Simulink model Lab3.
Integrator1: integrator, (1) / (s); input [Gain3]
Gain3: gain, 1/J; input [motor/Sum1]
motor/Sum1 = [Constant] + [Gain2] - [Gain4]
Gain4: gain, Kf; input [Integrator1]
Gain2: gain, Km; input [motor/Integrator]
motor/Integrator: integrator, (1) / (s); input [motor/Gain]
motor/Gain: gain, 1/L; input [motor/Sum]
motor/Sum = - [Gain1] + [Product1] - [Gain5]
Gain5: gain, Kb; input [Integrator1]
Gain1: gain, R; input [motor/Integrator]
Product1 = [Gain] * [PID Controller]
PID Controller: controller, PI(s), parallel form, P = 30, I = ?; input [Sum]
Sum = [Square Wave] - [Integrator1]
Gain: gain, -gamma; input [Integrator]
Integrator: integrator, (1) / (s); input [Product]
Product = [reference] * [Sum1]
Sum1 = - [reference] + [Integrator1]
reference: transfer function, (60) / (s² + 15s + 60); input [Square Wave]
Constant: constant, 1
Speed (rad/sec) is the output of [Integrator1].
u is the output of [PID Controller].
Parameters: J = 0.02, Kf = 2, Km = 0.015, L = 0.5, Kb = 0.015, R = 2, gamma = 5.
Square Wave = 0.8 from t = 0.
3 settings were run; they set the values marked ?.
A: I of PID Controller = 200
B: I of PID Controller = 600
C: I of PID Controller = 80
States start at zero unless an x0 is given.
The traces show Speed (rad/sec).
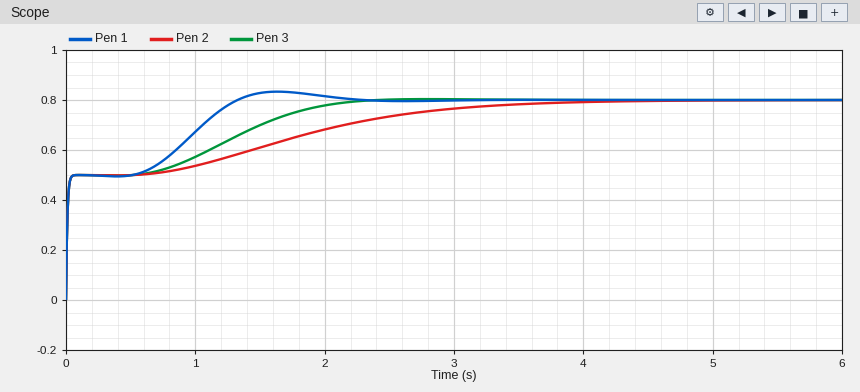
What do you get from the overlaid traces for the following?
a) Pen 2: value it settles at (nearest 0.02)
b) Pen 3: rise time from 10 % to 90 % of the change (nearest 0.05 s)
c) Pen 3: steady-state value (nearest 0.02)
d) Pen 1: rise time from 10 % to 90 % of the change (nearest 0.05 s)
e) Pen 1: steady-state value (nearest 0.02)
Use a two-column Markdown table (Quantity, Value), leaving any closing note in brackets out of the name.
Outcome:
| Quantity | Value |
|---|---|
| Pen 2: value it settles at | 0.80 |
| Pen 3: rise time from 10 % to 90 % of the change | 1.60 s |
| Pen 3: steady-state value | 0.80 |
| Pen 1: rise time from 10 % to 90 % of the change | 1.10 s |
| Pen 1: steady-state value | 0.80 |
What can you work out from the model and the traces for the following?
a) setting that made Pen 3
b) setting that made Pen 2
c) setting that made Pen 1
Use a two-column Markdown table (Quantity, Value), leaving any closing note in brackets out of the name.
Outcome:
| Quantity | Value |
|---|---|
| setting that made Pen 3 | A |
| setting that made Pen 2 | C |
| setting that made Pen 1 | B |
